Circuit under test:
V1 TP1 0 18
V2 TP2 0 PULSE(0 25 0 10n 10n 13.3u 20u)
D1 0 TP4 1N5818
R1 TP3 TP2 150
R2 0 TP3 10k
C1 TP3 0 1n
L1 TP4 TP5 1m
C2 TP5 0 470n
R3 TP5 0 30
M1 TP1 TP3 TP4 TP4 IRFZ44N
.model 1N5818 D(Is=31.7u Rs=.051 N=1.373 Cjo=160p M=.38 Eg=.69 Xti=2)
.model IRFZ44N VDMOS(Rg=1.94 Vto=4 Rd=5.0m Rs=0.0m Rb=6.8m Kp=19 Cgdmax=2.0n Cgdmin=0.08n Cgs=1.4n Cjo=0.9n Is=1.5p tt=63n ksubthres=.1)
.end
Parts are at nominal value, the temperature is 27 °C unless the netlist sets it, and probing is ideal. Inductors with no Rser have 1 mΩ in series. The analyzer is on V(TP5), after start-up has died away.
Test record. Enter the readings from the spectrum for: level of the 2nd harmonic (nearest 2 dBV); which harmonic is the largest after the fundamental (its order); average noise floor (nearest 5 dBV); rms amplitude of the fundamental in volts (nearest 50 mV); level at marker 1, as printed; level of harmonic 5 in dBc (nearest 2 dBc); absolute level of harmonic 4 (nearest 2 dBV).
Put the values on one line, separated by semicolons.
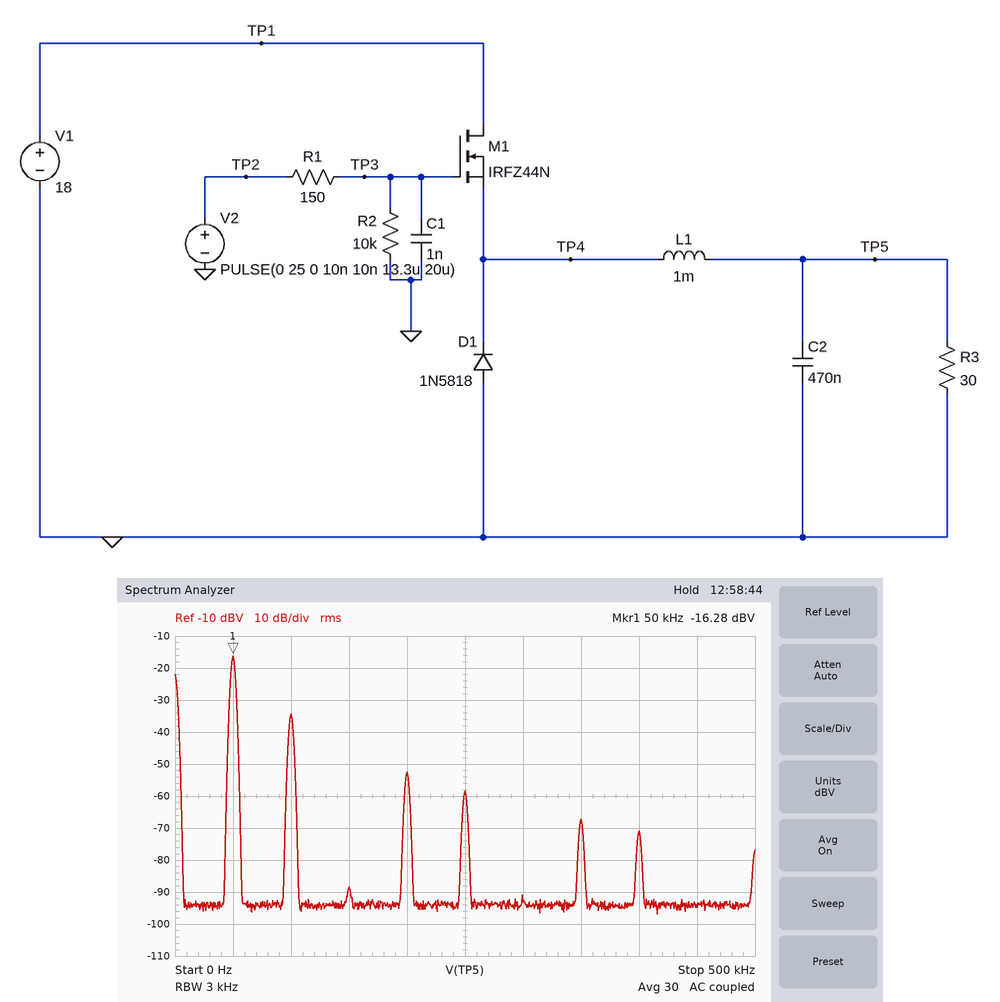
-34 dBV; 2; -95 dBV; 150 mV; -16.28 dBV; -42 dBc; -52 dBV
